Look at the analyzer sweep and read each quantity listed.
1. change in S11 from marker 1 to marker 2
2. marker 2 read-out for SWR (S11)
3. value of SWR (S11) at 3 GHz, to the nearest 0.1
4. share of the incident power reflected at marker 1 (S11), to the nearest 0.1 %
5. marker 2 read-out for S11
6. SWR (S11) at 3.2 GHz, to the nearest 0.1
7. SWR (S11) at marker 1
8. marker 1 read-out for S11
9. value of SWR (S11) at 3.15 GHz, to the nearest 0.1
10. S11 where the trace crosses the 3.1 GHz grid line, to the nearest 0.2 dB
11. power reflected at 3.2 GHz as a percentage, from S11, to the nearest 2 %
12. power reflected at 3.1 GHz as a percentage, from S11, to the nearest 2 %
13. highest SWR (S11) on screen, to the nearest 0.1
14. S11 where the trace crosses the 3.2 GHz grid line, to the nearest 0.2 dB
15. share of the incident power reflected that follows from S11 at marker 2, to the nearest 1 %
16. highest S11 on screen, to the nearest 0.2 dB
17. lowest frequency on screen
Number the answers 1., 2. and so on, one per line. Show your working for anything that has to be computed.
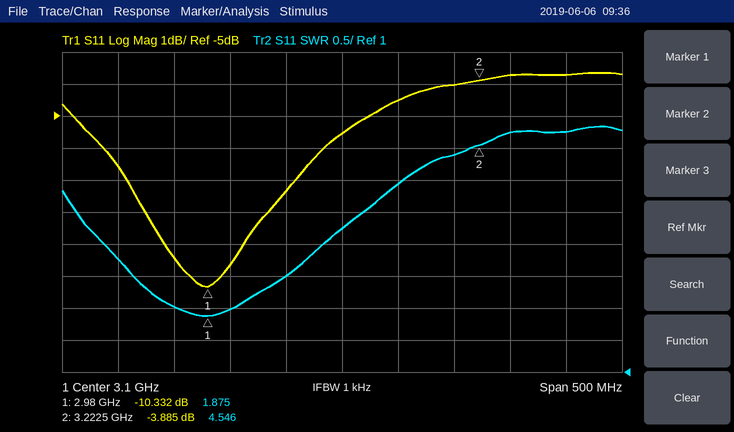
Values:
1. -3.885 − (-10.332) = 6.447 dB
2. 4.546
3. 2.0
4. 10^(-10.332/10) ≈ 9.3 %
5. -3.885 dB
6. 4.4
7. 1.875
8. -10.332 dB
9. 3.9
10. -5.6 dB
11. 10^(-4/10) ≈ 40 %
12. 10^(-5.6/10) ≈ 28 %
13. 4.8
14. -4.0 dB
15. 10^(-3.885/10) ≈ 41 %
16. -3.6 dB
17. 2.85 GHz
